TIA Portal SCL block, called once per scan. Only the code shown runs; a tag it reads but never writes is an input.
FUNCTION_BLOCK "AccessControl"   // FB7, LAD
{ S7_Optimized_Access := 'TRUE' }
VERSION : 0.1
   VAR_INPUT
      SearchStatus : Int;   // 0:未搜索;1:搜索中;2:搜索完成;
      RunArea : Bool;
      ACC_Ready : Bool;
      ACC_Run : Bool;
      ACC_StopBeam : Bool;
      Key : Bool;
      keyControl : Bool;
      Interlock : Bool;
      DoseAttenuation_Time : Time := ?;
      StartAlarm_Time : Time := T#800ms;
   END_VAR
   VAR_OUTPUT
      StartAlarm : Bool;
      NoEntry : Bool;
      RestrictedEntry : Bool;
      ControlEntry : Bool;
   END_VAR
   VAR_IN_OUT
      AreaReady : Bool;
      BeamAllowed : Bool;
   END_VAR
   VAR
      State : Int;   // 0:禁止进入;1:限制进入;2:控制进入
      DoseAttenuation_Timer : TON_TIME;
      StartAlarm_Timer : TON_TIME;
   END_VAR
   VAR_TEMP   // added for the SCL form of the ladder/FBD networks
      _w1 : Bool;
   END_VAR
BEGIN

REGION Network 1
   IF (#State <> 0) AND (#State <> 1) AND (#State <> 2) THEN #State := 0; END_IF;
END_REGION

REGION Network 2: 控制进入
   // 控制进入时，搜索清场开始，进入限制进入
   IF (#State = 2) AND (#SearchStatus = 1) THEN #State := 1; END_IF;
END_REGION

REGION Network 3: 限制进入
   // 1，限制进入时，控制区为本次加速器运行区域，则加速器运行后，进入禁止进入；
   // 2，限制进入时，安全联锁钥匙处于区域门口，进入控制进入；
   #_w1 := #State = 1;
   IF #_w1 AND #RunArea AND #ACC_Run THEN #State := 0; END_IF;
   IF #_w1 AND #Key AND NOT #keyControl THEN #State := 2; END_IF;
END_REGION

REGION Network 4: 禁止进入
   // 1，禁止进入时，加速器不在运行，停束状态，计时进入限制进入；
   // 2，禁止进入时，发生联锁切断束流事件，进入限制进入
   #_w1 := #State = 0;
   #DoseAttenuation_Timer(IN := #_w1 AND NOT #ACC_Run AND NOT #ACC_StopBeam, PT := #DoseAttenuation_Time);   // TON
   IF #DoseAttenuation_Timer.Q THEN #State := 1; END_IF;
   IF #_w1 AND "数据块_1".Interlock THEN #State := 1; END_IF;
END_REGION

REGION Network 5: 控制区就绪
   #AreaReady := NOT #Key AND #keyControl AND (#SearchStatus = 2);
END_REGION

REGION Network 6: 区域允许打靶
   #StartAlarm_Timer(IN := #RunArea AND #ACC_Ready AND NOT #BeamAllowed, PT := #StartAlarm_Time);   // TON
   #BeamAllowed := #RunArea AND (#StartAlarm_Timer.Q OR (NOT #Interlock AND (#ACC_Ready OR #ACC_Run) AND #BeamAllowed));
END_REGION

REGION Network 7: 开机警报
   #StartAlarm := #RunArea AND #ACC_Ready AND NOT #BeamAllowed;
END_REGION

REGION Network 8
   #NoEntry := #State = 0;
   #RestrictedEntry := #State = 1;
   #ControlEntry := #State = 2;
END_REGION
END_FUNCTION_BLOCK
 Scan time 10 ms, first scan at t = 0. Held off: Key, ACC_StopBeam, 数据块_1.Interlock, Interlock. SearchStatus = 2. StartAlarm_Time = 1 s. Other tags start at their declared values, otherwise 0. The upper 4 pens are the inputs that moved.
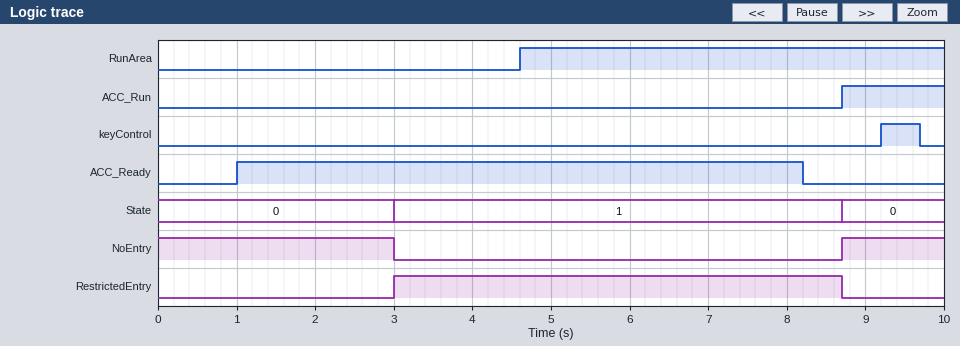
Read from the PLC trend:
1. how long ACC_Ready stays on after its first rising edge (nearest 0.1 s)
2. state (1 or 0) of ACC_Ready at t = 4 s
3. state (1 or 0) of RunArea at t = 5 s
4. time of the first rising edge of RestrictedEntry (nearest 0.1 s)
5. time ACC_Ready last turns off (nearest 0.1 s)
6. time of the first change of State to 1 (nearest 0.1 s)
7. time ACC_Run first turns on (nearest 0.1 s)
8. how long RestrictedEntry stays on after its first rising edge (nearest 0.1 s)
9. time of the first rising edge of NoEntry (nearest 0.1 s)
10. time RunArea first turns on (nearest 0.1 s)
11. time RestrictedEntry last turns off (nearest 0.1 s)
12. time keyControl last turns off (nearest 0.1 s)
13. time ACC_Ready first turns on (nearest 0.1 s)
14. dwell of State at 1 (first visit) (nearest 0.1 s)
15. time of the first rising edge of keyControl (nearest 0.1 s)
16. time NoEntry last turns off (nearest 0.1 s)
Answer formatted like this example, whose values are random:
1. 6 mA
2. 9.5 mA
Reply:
1. 7.2 s
2. 1
3. 1
4. 3.0 s
5. 8.2 s
6. 3.0 s
7. 8.7 s
8. 5.7 s
9. 8.7 s
10. 4.6 s
11. 8.7 s
12. 9.7 s
13. 1.0 s
14. 5.7 s
15. 9.2 s
16. 3.0 s
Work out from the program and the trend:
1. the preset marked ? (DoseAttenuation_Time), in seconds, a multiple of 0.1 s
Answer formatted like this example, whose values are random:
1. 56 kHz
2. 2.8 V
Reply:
1. 3.0 s
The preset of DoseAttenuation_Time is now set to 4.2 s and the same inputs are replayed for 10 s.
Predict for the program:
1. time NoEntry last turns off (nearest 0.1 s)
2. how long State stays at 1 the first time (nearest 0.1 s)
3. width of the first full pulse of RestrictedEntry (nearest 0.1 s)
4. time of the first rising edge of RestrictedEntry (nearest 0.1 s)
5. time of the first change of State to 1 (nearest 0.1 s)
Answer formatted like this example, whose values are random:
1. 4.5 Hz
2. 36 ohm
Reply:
1. 4.2 s
2. 4.5 s
3. 4.5 s
4. 4.2 s
5. 4.2 s
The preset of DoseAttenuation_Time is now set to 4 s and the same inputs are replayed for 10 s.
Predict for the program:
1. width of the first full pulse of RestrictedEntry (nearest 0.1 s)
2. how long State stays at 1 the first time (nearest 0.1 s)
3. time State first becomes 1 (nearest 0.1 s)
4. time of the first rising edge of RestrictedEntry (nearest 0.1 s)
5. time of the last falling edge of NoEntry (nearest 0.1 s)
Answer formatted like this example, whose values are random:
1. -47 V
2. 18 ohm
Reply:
1. 4.7 s
2. 4.7 s
3. 4.0 s
4. 4.0 s
5. 4.0 s
